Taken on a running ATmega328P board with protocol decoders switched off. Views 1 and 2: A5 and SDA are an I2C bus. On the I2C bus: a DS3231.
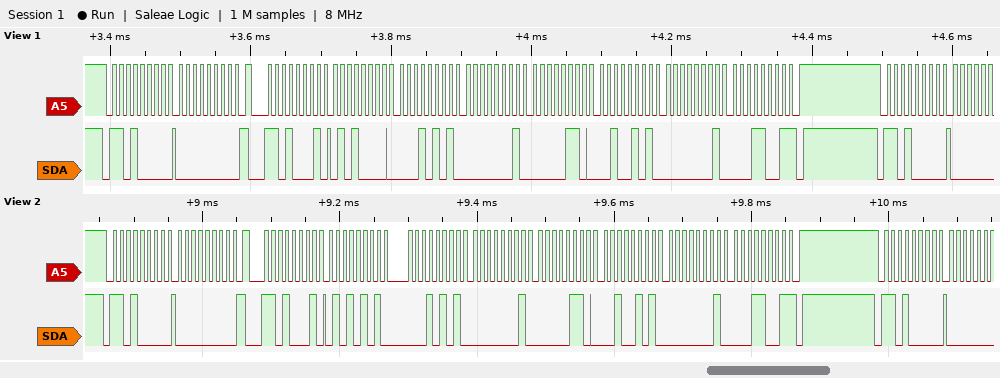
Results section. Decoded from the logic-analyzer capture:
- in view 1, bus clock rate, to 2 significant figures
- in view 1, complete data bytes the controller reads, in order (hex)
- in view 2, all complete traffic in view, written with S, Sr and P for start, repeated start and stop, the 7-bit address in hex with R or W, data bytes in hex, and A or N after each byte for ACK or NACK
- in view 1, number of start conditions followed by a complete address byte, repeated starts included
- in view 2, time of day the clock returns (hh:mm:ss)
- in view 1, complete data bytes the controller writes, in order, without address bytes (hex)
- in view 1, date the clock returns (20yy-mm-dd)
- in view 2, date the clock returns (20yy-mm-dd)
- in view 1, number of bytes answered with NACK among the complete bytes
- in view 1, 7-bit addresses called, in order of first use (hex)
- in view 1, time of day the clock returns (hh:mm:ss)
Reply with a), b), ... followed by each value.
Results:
a) 100 kHz
b) 50 15 01 06 25 01 19
c) S 68W A 00 A Sr 68R A 55 A 15 A 01 A 06 A 25 A 01 A 19 N P S 68W A
d) 3
e) 01:15:55
f) 00
g) 2019-01-25
h) 2019-01-25
i) 1
j) 0x68
k) 01:15:50
